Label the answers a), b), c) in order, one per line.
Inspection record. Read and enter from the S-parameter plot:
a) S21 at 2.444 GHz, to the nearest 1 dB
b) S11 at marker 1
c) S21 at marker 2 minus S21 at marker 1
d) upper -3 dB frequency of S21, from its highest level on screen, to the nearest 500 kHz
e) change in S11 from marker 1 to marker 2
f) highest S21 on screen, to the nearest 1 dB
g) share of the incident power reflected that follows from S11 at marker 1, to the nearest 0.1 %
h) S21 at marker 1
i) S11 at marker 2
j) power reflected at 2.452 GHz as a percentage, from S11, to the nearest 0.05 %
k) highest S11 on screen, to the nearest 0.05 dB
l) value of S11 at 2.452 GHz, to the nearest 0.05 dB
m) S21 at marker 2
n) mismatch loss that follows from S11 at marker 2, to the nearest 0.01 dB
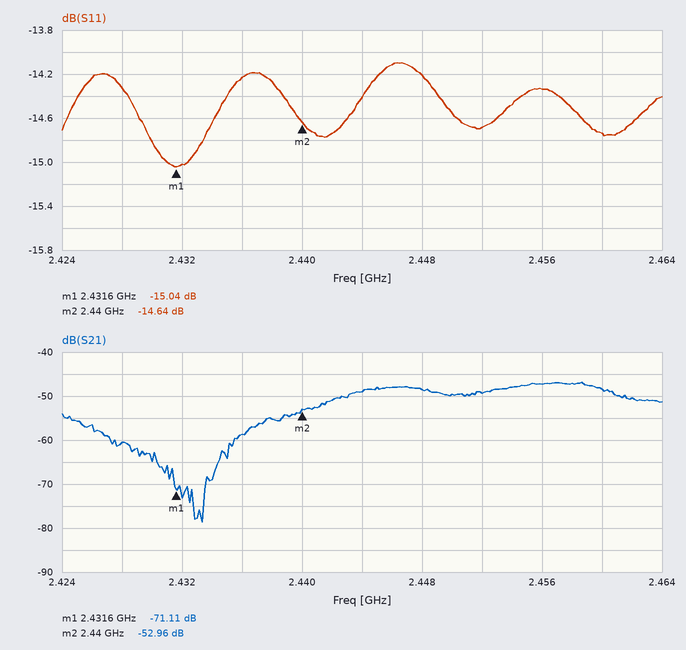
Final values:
a) -49 dB
b) -15.04 dB
c) 18.15 dB
d) 2.4610 GHz
e) 0.40 dB
f) -47 dB
g) 3.1 %
h) -71.11 dB
i) -14.64 dB
j) 3.40 %
k) -14.10 dB
l) -14.70 dB
m) -52.96 dB
n) 0.15 dB
